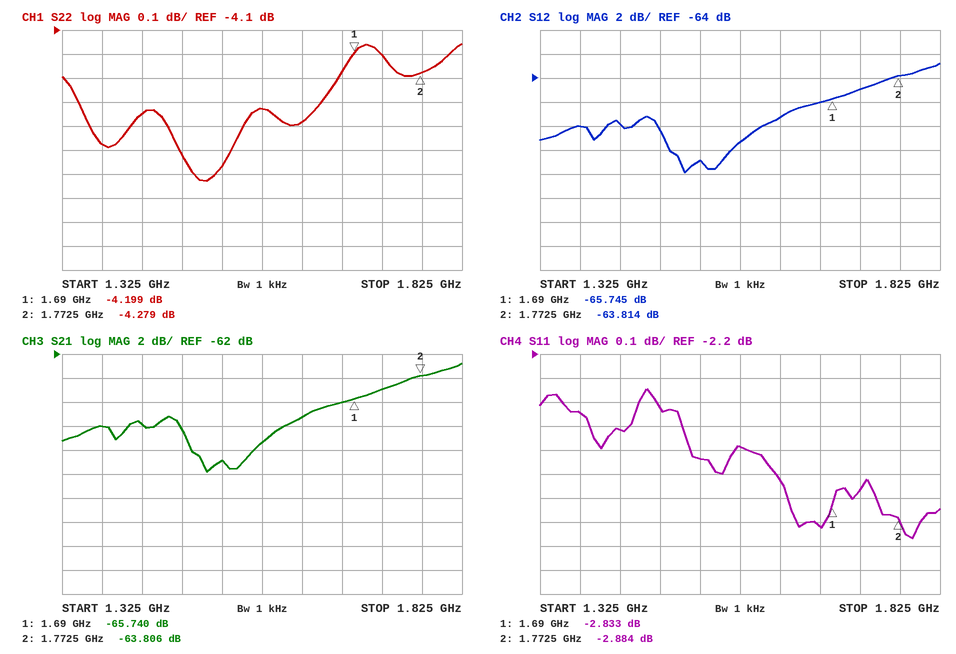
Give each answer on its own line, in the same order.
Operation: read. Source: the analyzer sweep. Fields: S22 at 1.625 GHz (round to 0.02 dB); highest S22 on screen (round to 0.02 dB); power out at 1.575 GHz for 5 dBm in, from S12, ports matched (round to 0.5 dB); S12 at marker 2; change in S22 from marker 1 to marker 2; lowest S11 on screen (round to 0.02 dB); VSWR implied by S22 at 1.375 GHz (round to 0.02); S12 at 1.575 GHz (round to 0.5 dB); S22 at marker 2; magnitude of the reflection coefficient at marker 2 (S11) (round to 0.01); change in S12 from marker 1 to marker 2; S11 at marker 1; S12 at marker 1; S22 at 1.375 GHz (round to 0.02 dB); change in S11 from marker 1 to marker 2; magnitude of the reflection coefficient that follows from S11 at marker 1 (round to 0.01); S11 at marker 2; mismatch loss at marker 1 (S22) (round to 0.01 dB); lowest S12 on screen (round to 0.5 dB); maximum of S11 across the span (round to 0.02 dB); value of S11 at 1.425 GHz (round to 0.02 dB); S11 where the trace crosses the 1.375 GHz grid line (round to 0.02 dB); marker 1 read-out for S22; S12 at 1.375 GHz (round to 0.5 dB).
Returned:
-4.48 dB
-4.16 dB
-64.5 dBm
-63.814 dB
-0.080 dB
-2.96 dB
3.88
-69.5 dB
-4.279 dB
0.72
1.931 dB
-2.833 dB
-65.745 dB
-4.58 dB
-0.051 dB
0.72
-2.884 dB
2.08 dB
-72.0 dB
-2.34 dB
-2.52 dB
-2.44 dB
-4.199 dB
-68.0 dB
